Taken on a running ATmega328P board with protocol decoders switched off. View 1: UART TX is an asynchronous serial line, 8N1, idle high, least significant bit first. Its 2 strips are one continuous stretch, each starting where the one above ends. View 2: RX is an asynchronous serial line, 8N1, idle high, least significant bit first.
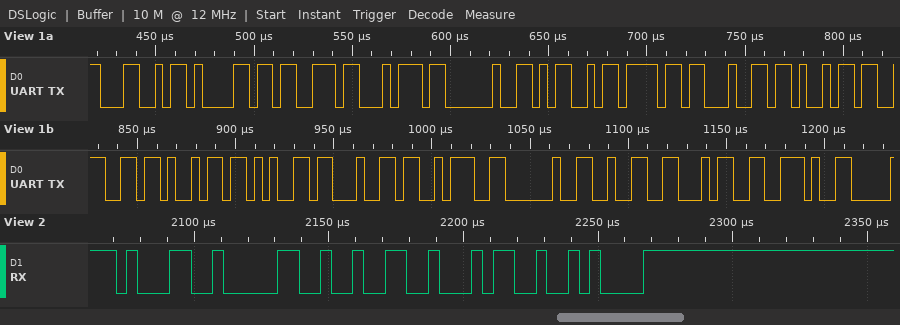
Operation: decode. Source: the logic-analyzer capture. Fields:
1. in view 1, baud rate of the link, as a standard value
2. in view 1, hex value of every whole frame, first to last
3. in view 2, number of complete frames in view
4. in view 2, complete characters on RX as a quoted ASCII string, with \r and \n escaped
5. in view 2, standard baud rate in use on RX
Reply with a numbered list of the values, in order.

1. 250000 baud
2. 0x4C 0x61 0x73 0x74 0x20 0x4D 0x6F 0x64 0x69 0x66 0x69 0x65 0x64 0x3A 0x20 0x32 0x34 0x2E
3. 5
4. "1024\n"
5. 250000 baud
